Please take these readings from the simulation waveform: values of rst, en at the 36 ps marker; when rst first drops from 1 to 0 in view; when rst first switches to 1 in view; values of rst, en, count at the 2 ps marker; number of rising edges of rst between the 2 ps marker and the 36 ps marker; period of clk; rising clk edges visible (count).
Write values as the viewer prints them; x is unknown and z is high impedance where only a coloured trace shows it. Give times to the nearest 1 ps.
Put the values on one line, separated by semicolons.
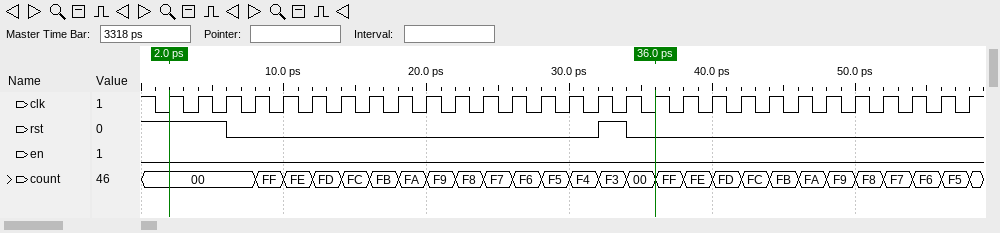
rst=0, en=0; 6 ps; 32 ps; rst=1, en=0, count=00; 1; 2 ps; 29
